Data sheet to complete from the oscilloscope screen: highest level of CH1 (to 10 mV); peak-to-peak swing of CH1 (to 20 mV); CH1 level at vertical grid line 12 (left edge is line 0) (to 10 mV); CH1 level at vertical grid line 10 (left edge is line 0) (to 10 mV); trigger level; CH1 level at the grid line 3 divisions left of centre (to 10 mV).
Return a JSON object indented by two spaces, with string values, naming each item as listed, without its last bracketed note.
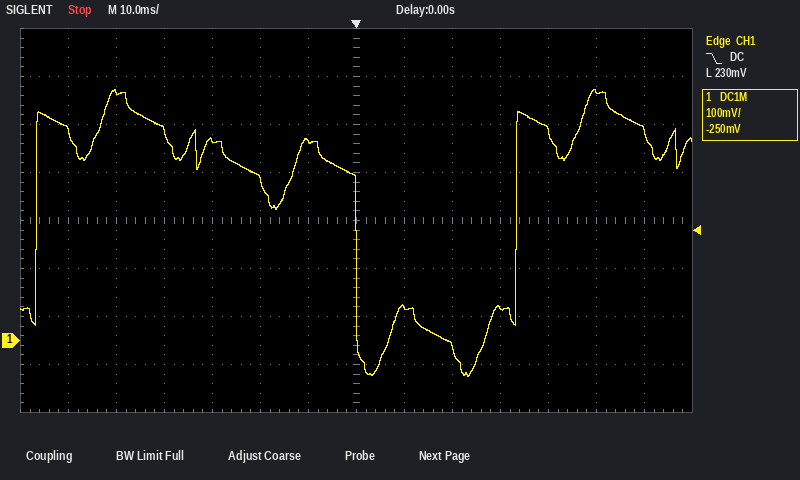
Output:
{
  "highest level of CH1": "520 mV",
  "peak-to-peak swing of CH1": "600 mV",
  "CH1 level at vertical grid line 12 (left edge is line 0)": "520 mV",
  "CH1 level at vertical grid line 10 (left edge is line 0)": "70 mV",
  "trigger level": "230 mV",
  "CH1 level at the grid line 3 divisions left of centre": "420 mV"
}
